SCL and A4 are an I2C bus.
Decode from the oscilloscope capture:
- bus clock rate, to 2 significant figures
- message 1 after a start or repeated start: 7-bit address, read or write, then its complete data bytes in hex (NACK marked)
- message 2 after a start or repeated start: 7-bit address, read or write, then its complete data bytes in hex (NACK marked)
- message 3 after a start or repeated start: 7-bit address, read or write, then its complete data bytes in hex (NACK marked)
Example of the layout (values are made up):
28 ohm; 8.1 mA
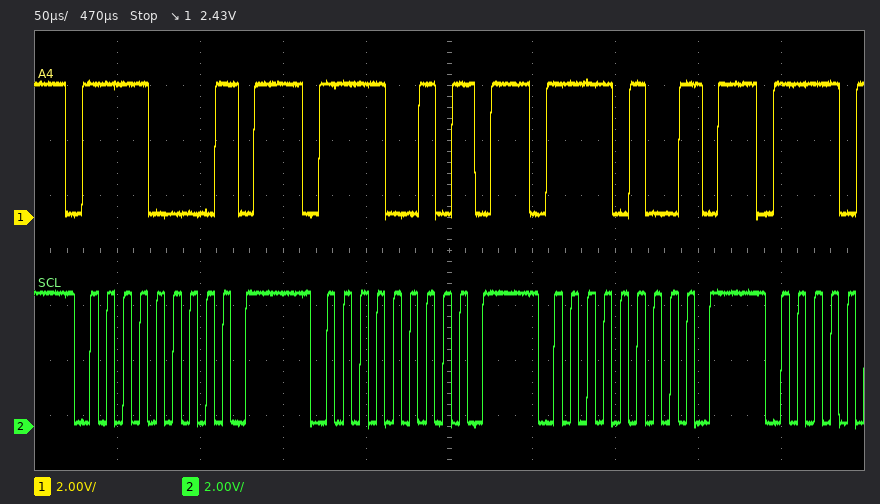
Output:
100 kHz; 0x78 write NACK; 0x79 write NACK; 0x7A write NACK
